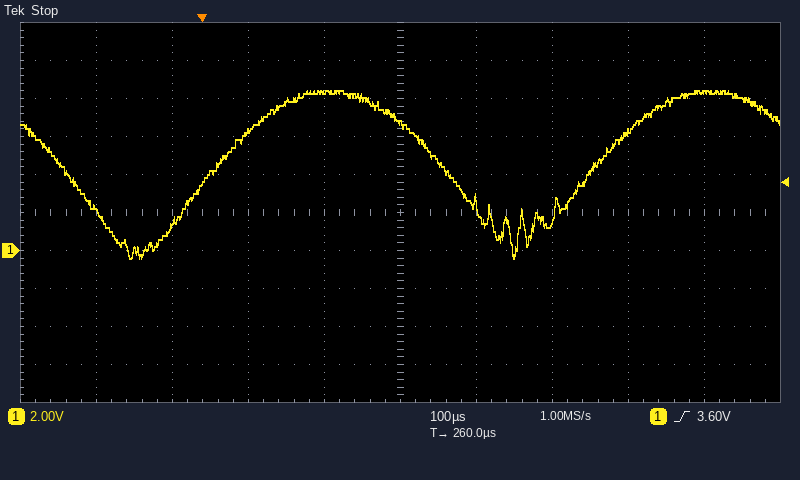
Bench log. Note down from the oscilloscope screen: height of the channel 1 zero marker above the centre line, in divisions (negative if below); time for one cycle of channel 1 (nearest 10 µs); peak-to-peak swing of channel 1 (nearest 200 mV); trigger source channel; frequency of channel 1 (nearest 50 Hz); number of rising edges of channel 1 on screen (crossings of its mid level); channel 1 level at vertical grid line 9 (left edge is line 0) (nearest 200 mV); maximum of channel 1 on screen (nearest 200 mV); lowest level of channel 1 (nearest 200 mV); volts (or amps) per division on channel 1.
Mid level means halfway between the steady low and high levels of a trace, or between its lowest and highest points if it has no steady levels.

-1.0 div
500 µs
8.8 V
channel 1
2.00 kHz
2
8.4 V
8.4 V
-400 mV
2 V
